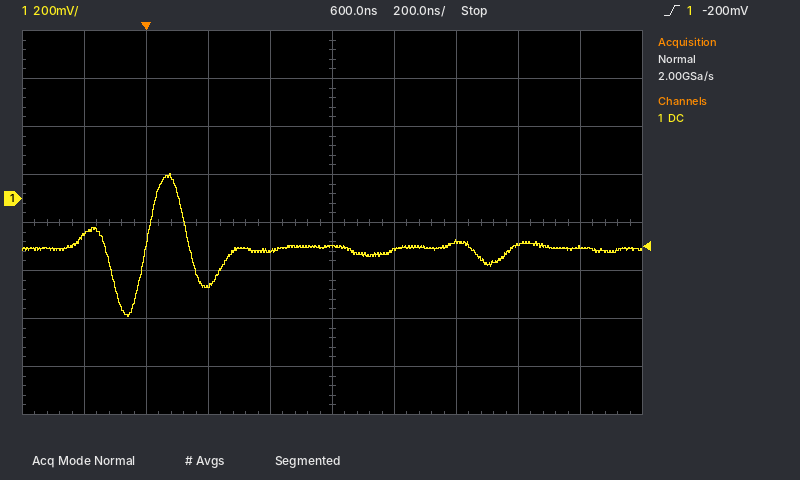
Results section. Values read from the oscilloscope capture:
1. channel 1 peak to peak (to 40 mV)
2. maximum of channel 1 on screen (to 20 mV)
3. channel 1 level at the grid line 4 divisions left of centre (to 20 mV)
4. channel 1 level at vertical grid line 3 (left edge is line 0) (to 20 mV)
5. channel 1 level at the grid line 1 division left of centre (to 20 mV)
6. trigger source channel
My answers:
600 mV
100 mV
-160 mV
-360 mV
-220 mV
channel 1
